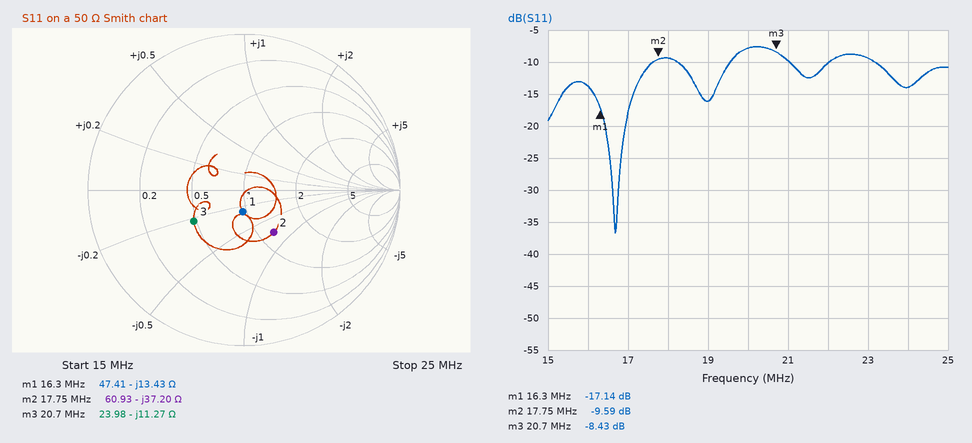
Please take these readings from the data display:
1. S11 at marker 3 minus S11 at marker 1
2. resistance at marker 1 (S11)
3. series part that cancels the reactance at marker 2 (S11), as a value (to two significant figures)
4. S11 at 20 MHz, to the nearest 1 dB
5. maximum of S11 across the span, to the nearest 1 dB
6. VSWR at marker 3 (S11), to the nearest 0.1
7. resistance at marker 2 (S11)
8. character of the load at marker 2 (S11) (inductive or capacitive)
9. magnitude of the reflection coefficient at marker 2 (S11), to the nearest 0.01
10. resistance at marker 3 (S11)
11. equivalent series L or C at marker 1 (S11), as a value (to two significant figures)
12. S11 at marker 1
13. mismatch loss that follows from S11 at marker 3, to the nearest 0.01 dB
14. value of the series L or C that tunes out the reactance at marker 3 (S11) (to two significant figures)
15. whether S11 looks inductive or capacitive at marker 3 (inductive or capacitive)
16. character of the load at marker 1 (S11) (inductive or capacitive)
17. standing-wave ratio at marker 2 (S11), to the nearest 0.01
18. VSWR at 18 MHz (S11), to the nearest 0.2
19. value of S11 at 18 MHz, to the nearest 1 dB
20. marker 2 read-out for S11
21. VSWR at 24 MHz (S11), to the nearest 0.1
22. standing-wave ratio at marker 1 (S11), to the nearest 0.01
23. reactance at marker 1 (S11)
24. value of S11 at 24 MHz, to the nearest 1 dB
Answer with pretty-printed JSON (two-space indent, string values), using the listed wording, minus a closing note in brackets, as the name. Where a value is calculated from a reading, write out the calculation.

{
  "S11 at marker 3 minus S11 at marker 1": "-8.43 − (-17.14) = 8.71 dB",
  "resistance at marker 1": "47.41 Ω",
  "series part that cancels the reactance at marker 2 (S11), as a value": "L = 37.2 Ω/(2π × 17.75 MHz) ≈ 334 nH, so 330 nH to two significant figures",
  "S11 at 20 MHz, to the nearest 1 dB": "-8 dB",
  "maximum of S11 across the span, to the nearest 1 dB": "-8 dB",
  "VSWR at marker 3 (S11), to the nearest 0.1": "2.2",
  "resistance at marker 2": "60.93 Ω",
  "character of the load at marker 2 (S11)": "capacitive",
  "magnitude of the reflection coefficient at marker 2 (S11), to the nearest 0.01": "10^(-9.59/20) ≈ 0.33",
  "resistance at marker 3": "23.98 Ω",
  "equivalent series L or C at marker 1 (S11), as a value": "C = 1/(2π × 16.3 MHz × 13.43 Ω) ≈ 727 pF, so 730 pF to two significant figures",
  "S11 at marker 1": "-17.14 dB",
  "mismatch loss that follows from S11 at marker 3, to the nearest 0.01 dB": "−10 log10(1 − 10^(-8.43/10)) ≈ 0.67 dB",
  "value of the series L or C that tunes out the reactance at marker 3 (S11)": "L = 11.27 Ω/(2π × 20.7 MHz) ≈ 87 nH",
  "whether S11 looks inductive or capacitive at marker 3": "capacitive",
  "character of the load at marker 1 (S11)": "capacitive",
  "standing-wave ratio at marker 2 (S11), to the nearest 0.01": "1.99",
  "VSWR at 18 MHz (S11), to the nearest 0.2": "|Γ| = 10^(-9/20) = 0.3548; VSWR = (1 + 0.3548)/(1 − 0.3548) ≈ 2.10, so 2.0 to the nearest 0.2",
  "value of S11 at 18 MHz, to the nearest 1 dB": "-9 dB",
  "marker 2 read-out for S11": "-9.59 dB",
  "VSWR at 24 MHz (S11), to the nearest 0.1": "|Γ| = 10^(-14/20) = 0.1995; VSWR = (1 + 0.1995)/(1 − 0.1995) ≈ 1.5",
  "standing-wave ratio at marker 1 (S11), to the nearest 0.01": "1.32",
  "reactance at marker 1": "-13.43 Ω",
  "value of S11 at 24 MHz, to the nearest 1 dB": "-14 dB"
}
